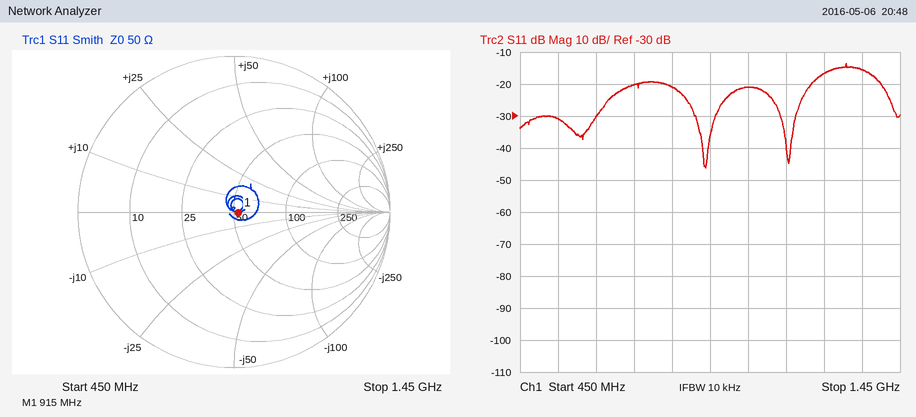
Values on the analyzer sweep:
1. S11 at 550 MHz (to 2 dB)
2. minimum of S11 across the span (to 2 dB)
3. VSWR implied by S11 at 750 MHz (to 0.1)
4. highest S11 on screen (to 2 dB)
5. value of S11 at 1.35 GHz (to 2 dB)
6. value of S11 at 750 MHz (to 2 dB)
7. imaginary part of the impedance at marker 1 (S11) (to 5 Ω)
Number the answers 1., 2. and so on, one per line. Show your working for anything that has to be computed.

1. -30 dB
2. -46 dB
3. |Γ| = 10^(-20/20) = 0.1000; VSWR = (1 + 0.1000)/(1 − 0.1000) ≈ 1.2
4. -14 dB
5. -16 dB
6. -20 dB
7. 0 Ω
